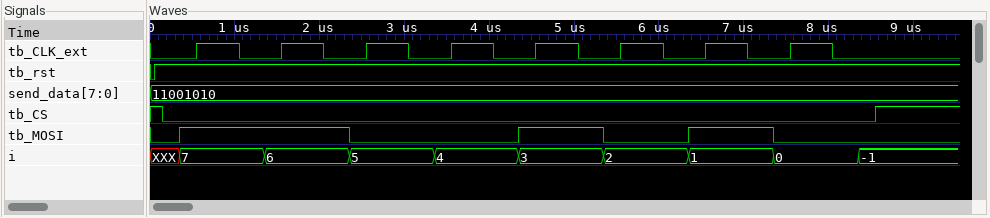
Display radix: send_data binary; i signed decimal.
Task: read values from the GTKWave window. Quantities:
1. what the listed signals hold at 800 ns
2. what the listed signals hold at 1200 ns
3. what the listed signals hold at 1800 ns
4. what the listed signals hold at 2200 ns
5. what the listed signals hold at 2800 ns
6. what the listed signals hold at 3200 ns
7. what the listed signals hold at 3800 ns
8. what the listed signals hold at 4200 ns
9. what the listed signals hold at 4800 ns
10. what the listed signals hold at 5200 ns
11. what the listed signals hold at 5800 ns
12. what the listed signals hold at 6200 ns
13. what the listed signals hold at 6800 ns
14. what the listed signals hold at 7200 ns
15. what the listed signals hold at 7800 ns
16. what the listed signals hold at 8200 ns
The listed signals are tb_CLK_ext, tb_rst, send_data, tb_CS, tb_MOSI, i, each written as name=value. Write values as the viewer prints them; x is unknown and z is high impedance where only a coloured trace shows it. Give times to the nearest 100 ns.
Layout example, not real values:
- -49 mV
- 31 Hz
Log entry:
- tb_CLK_ext=1, tb_rst=1, send_data=11001010, tb_CS=0, tb_MOSI=1, i=7
- tb_CLK_ext=0, tb_rst=1, send_data=11001010, tb_CS=0, tb_MOSI=1, i=7
- tb_CLK_ext=1, tb_rst=1, send_data=11001010, tb_CS=0, tb_MOSI=1, i=6
- tb_CLK_ext=0, tb_rst=1, send_data=11001010, tb_CS=0, tb_MOSI=1, i=6
- tb_CLK_ext=1, tb_rst=1, send_data=11001010, tb_CS=0, tb_MOSI=0, i=5
- tb_CLK_ext=0, tb_rst=1, send_data=11001010, tb_CS=0, tb_MOSI=0, i=5
- tb_CLK_ext=1, tb_rst=1, send_data=11001010, tb_CS=0, tb_MOSI=0, i=4
- tb_CLK_ext=0, tb_rst=1, send_data=11001010, tb_CS=0, tb_MOSI=0, i=4
- tb_CLK_ext=1, tb_rst=1, send_data=11001010, tb_CS=0, tb_MOSI=1, i=3
- tb_CLK_ext=0, tb_rst=1, send_data=11001010, tb_CS=0, tb_MOSI=1, i=3
- tb_CLK_ext=1, tb_rst=1, send_data=11001010, tb_CS=0, tb_MOSI=0, i=2
- tb_CLK_ext=0, tb_rst=1, send_data=11001010, tb_CS=0, tb_MOSI=0, i=2
- tb_CLK_ext=1, tb_rst=1, send_data=11001010, tb_CS=0, tb_MOSI=1, i=1
- tb_CLK_ext=0, tb_rst=1, send_data=11001010, tb_CS=0, tb_MOSI=1, i=1
- tb_CLK_ext=1, tb_rst=1, send_data=11001010, tb_CS=0, tb_MOSI=0, i=0
- tb_CLK_ext=0, tb_rst=1, send_data=11001010, tb_CS=0, tb_MOSI=0, i=0
